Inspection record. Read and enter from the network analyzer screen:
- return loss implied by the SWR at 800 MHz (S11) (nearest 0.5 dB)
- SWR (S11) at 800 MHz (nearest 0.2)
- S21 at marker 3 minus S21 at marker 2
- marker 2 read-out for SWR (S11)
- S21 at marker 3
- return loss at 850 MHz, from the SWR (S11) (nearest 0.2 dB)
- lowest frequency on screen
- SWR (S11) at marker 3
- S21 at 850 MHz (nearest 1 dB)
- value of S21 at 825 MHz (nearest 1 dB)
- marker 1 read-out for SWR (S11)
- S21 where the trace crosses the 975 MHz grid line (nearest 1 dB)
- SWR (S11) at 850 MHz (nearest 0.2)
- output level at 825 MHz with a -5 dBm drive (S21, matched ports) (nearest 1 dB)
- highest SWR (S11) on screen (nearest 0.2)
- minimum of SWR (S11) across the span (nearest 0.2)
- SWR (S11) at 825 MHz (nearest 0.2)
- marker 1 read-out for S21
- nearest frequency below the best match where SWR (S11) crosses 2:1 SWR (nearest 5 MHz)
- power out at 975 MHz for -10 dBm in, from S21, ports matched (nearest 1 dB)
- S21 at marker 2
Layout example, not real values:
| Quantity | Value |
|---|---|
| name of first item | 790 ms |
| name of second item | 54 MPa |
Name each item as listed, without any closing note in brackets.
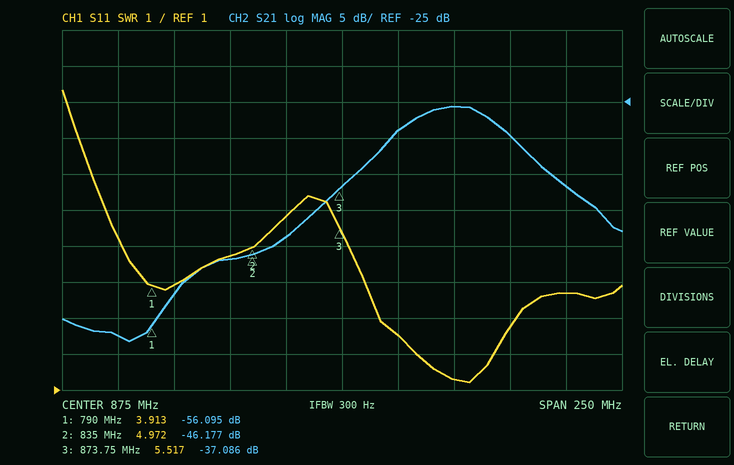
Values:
| Quantity | Value |
|---|---|
| return loss implied by the SWR at 800 MHz (S11) | 4.5 dB |
| SWR (S11) at 800 MHz | 4.0 |
| S21 at marker 3 minus S21 at marker 2 | 9.091 dB |
| marker 2 read-out for SWR | 4.972 |
| S21 at marker 3 | -37.086 dB |
| return loss at 850 MHz, from the SWR (S11) | 3.0 dB |
| lowest frequency on screen | 750 MHz |
| SWR (S11) at marker 3 | 5.517 |
| S21 at 850 MHz | -44 dB |
| value of S21 at 825 MHz | -47 dB |
| marker 1 read-out for SWR | 3.913 |
| S21 where the trace crosses the 975 MHz grid line | -37 dB |
| SWR (S11) at 850 MHz | 5.8 |
| output level at 825 MHz with a -5 dBm drive (S21, matched ports) | -52 dBm |
| highest SWR (S11) on screen | 9.4 |
| minimum of SWR (S11) across the span | 1.2 |
| SWR (S11) at 825 MHz | 4.8 |
| marker 1 read-out for S21 | -56.095 dB |
| nearest frequency below the best match where SWR (S11) crosses 2:1 SWR | 910 MHz |
| power out at 975 MHz for -10 dBm in, from S21, ports matched | -47 dBm |
| S21 at marker 2 | -46.177 dB |
